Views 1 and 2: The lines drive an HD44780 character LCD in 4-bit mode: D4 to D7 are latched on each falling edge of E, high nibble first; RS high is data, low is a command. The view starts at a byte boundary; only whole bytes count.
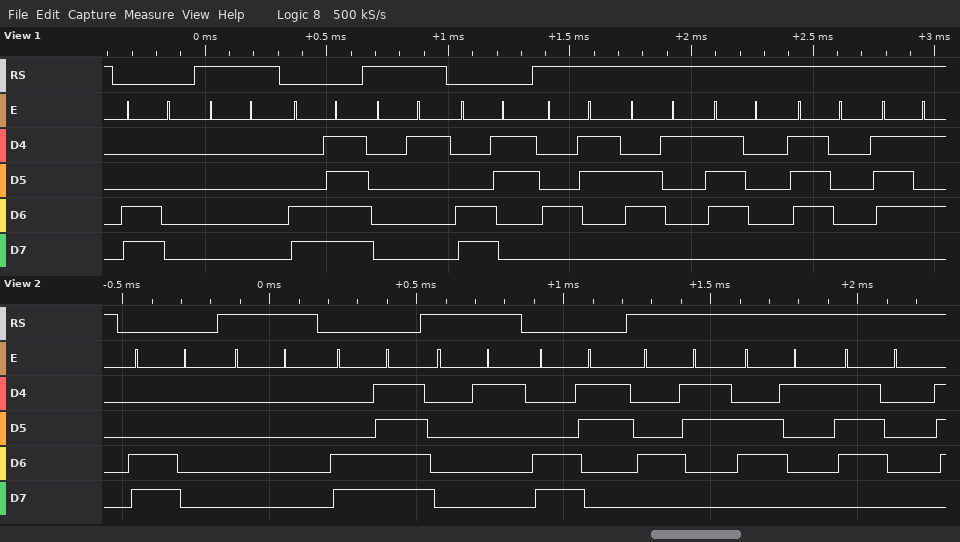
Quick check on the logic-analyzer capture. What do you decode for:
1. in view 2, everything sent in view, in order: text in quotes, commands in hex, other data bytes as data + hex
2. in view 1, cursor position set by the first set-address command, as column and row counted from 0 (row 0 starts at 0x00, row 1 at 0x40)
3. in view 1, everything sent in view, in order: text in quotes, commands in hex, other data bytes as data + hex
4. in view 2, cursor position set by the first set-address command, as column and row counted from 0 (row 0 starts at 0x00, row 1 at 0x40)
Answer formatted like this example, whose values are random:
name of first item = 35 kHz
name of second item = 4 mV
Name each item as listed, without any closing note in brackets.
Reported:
in view 2, everything sent in view, in order: text in quotes, commands in hex, other data bytes as data + hex = 0xC0 data 00 0xCF data 01 0xC3 "Cap"
in view 1, cursor position set by the first set-address command, as column and row counted from 0 = column 0, row 1
in view 1, everything sent in view, in order: text in quotes, commands in hex, other data bytes as data + hex = 0xC0 data 00 0xCF data 01 0xC3 "Cappu"
in view 2, cursor position set by the first set-address command, as column and row counted from 0 = column 0, row 1
